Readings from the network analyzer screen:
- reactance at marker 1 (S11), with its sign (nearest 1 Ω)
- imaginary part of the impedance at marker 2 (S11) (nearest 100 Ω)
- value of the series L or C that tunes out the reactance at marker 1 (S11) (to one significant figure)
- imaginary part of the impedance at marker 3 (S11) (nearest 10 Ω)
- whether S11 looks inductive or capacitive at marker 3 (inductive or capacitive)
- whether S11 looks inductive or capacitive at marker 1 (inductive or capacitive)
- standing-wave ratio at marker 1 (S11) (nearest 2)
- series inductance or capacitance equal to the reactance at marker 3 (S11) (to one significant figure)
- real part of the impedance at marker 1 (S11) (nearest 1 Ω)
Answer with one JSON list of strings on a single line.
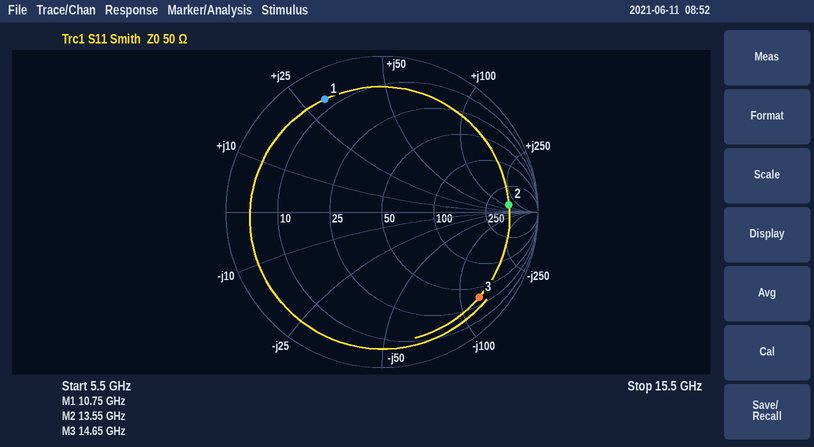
["+30 Ω", "+100 Ω", "500 fF", "-120 Ω", "capacitive", "inductive", "10", "90 fF", "7 Ω"]
